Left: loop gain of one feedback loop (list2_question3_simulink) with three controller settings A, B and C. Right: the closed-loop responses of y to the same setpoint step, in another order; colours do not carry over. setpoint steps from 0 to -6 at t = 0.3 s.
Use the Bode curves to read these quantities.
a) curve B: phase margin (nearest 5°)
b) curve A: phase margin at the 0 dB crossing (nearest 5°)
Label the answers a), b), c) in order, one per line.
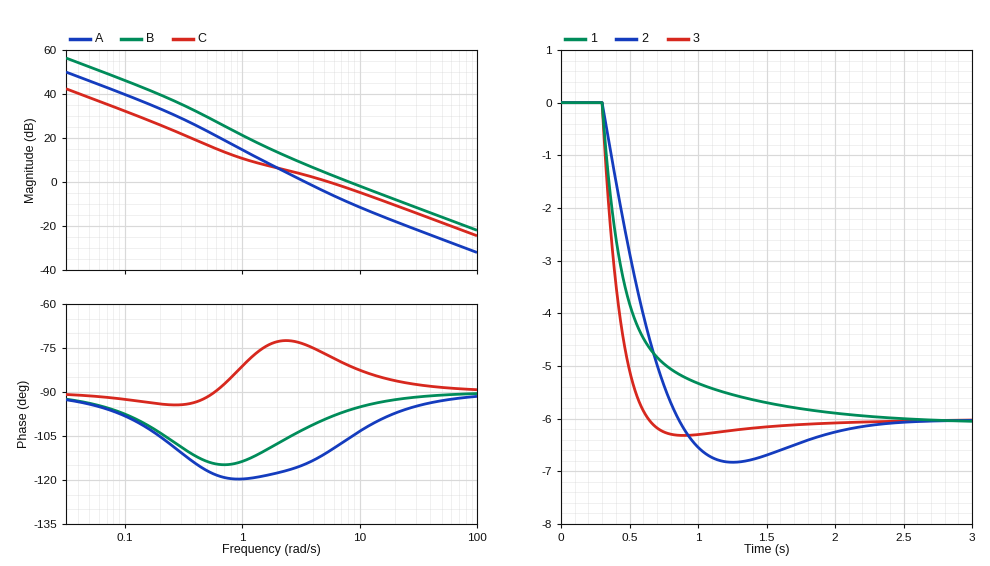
a) 85°
b) 65°
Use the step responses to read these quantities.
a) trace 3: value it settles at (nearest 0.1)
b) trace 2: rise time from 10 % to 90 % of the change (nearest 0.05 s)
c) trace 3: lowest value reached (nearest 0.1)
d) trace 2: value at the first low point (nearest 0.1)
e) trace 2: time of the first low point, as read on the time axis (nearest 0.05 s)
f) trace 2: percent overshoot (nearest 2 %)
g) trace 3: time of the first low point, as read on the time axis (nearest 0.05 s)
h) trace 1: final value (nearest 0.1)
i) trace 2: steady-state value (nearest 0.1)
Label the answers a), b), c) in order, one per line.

a) -6.0
b) 0.40 s
c) -6.3
d) -6.8
e) 1.25 s
f) 14 %
g) 0.90 s
h) -6.0
i) -6.0
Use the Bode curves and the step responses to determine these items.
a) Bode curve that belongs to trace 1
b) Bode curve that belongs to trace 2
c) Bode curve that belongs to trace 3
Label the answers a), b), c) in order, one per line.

a) C
b) A
c) B
